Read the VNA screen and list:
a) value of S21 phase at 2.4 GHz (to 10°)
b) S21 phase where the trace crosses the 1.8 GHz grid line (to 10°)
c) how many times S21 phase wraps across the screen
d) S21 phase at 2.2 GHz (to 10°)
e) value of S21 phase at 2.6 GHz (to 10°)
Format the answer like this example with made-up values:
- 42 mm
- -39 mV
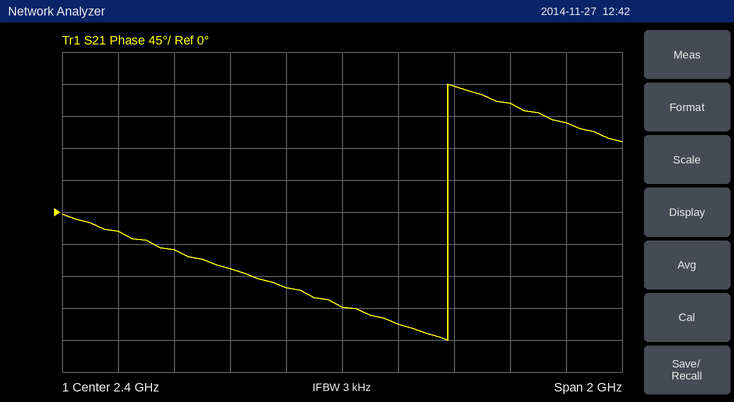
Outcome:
- -130°
- -50°
- 1
- -110°
- -160°
